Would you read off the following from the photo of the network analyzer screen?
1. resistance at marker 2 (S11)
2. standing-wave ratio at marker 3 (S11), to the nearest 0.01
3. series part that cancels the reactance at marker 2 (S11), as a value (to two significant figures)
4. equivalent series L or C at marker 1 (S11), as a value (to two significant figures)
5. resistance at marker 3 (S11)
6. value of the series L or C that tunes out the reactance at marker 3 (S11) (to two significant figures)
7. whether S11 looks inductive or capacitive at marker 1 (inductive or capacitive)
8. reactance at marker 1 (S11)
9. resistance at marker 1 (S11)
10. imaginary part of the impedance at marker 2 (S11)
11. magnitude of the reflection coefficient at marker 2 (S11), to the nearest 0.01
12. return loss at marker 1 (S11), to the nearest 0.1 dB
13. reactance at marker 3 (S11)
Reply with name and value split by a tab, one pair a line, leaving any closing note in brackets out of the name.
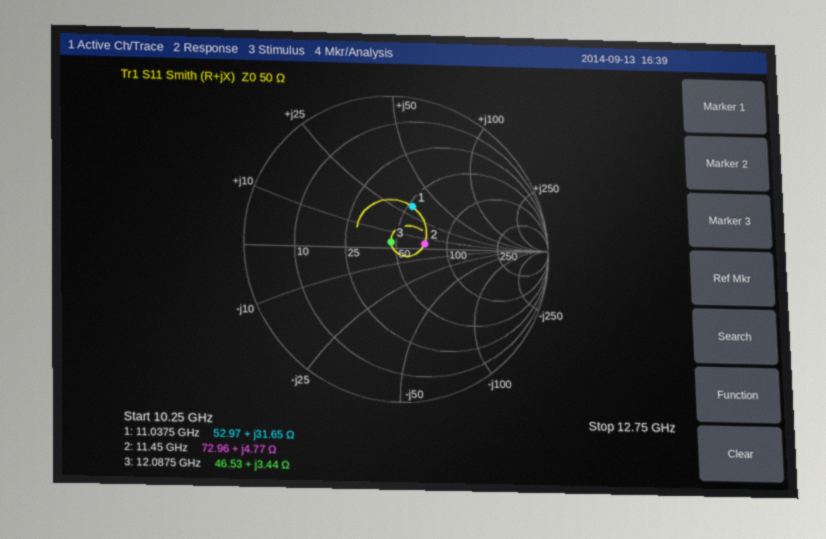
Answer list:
resistance at marker 2	72.96 Ω
standing-wave ratio at marker 3 (S11), to the nearest 0.01	1.11
series part that cancels the reactance at marker 2 (S11), as a value	2.9 pF
equivalent series L or C at marker 1 (S11), as a value	460 pH
resistance at marker 3	46.53 Ω
value of the series L or C that tunes out the reactance at marker 3 (S11)	3.8 pF
whether S11 looks inductive or capacitive at marker 1	inductive
reactance at marker 1	+31.65 Ω
resistance at marker 1	52.97 Ω
imaginary part of the impedance at marker 2	+4.77 Ω
magnitude of the reflection coefficient at marker 2 (S11), to the nearest 0.01	0.19
return loss at marker 1 (S11), to the nearest 0.1 dB	10.6 dB
reactance at marker 3	+3.44 Ω
